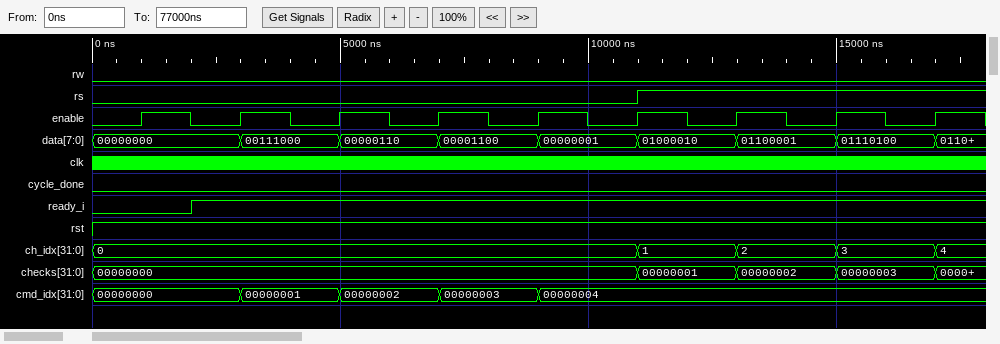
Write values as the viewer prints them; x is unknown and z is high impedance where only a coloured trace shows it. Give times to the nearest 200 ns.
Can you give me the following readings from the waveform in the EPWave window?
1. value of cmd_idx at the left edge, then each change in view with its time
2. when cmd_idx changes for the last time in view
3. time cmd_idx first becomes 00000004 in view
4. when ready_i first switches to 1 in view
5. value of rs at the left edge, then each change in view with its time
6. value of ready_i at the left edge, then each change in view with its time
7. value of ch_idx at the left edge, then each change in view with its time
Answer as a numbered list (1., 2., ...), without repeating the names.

1. 00000000, 00000001 at 3000 ns, 00000002 at 5000 ns, 00000003 at 7000 ns, 00000004 at 9000 ns
2. 9000 ns
3. 9000 ns
4. 2000 ns
5. 0, 1 at 11000 ns
6. 0, 1 at 2000 ns
7. 0, 1 at 11000 ns, 2 at 13000 ns, 3 at 15000 ns, 4 at 17000 ns
